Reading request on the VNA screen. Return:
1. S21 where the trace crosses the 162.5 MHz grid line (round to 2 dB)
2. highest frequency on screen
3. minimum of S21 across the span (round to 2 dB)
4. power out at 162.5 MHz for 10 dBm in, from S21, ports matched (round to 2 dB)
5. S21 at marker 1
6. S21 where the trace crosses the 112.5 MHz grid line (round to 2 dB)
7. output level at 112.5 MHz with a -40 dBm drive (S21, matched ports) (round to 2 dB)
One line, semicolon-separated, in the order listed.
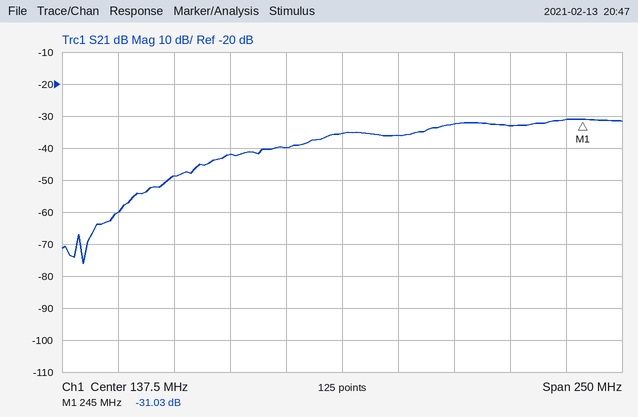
-36 dB; 262.5 MHz; -76 dB; -26 dBm; -31.03 dB; -40 dB; -80 dBm
